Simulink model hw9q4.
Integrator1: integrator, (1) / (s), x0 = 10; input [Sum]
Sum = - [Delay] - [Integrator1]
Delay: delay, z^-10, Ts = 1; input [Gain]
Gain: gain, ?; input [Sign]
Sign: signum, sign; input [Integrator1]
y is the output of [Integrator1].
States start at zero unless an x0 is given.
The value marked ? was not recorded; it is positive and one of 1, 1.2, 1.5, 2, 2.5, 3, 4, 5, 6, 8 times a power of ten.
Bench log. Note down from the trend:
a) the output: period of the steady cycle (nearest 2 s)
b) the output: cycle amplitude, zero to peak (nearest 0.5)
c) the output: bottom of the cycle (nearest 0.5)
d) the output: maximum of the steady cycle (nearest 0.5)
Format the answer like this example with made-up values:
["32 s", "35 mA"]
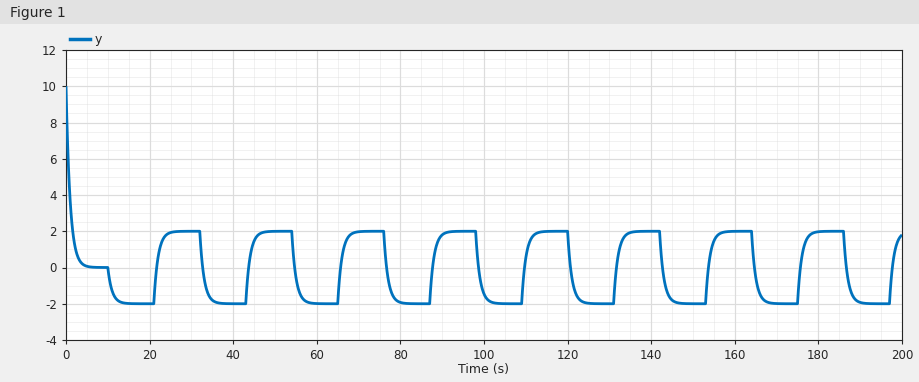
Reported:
["22 s", "2.0", "-2.0", "2.0"]
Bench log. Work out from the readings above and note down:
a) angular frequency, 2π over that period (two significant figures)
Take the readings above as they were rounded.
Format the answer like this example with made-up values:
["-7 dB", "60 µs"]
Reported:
["0.29 rad/s"]
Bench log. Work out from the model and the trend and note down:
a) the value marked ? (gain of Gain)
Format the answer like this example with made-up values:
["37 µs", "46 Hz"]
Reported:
["2"]
